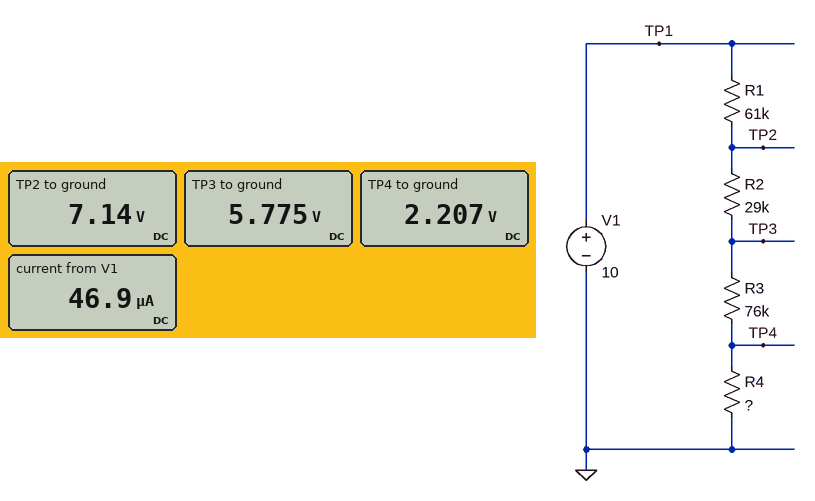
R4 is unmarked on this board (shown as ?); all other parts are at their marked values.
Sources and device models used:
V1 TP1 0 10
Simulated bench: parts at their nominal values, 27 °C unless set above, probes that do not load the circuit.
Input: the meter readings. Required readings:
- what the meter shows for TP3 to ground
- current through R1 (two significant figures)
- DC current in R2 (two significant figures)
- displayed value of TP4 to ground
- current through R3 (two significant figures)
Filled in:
5.775 V
47 µA
47 µA
2.207 V
47 µA
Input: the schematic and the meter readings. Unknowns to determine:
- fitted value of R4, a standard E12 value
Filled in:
47 kΩ
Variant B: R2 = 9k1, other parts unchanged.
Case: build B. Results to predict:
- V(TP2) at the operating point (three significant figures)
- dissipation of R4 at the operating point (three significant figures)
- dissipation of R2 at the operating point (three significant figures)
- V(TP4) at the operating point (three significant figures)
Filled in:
6.84 V
126 µW
24.4 µW
2.43 V
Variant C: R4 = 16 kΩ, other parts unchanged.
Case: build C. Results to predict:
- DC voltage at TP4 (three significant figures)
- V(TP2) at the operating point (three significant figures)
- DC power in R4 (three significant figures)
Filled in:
879 mV
6.65 V
48.3 µW
